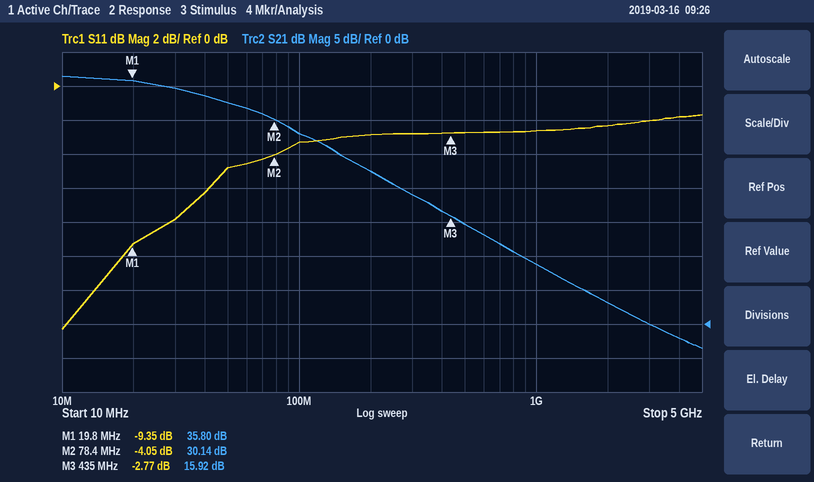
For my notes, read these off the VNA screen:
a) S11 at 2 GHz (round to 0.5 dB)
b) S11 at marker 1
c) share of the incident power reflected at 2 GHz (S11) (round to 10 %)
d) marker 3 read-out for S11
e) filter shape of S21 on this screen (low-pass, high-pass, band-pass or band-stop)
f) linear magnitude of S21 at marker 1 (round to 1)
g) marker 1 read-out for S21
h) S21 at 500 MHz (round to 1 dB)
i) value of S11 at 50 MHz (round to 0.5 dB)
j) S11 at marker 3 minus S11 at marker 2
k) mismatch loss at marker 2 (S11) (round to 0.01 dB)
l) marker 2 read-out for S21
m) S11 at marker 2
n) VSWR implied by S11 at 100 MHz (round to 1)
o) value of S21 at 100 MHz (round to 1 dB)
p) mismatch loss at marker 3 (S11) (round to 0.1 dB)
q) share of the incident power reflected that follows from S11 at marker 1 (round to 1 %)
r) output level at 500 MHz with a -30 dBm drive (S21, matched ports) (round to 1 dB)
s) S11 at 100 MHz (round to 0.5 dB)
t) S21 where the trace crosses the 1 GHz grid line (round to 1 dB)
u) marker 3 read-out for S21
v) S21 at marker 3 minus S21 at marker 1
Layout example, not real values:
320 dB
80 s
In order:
-2.5 dB
-9.35 dB
60 %
-2.77 dB
low-pass
62
35.80 dB
15 dB
-5.0 dB
1.28 dB
2.17 dB
30.14 dB
-4.05 dB
5
28 dB
3.3 dB
12 %
-15 dBm
-3.5 dB
9 dB
15.92 dB
-19.88 dB
